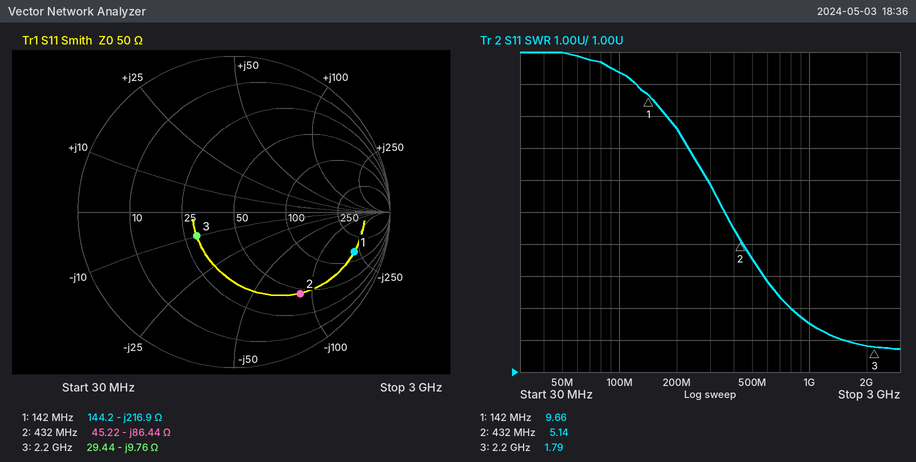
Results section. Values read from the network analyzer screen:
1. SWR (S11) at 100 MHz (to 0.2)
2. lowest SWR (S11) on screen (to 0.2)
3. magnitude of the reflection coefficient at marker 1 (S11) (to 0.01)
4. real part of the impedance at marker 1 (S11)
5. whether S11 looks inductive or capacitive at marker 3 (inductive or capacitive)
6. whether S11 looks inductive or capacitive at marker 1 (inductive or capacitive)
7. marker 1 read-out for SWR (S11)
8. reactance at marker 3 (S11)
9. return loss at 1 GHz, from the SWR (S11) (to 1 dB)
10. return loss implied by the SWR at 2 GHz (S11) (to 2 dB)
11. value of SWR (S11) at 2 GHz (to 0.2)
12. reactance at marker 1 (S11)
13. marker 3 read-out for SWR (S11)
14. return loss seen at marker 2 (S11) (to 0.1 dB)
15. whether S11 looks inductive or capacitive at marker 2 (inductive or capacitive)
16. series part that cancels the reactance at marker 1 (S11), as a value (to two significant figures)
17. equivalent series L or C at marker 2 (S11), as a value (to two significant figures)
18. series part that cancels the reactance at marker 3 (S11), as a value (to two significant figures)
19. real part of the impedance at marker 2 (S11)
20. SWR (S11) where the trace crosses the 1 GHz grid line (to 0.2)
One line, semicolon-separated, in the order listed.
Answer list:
10.4; 1.8; 0.81; 144.2 Ω; capacitive; capacitive; 9.66; -9.76 Ω; 7 dB; 10 dB; 1.8; -216.9 Ω; 1.79; 3.4 dB; capacitive; 240 nH; 4.3 pF; 710 pH; 45.22 Ω; 2.6
